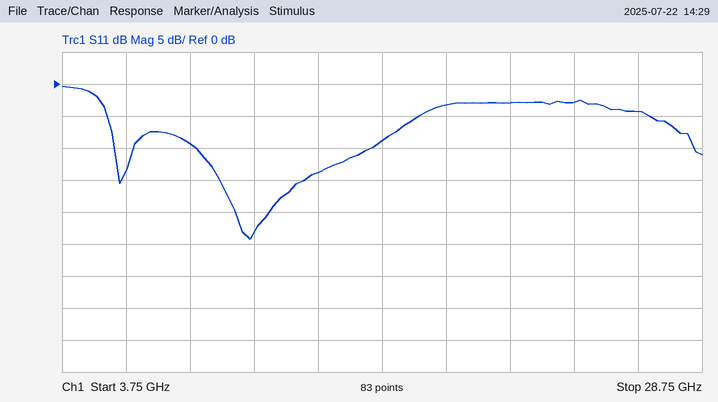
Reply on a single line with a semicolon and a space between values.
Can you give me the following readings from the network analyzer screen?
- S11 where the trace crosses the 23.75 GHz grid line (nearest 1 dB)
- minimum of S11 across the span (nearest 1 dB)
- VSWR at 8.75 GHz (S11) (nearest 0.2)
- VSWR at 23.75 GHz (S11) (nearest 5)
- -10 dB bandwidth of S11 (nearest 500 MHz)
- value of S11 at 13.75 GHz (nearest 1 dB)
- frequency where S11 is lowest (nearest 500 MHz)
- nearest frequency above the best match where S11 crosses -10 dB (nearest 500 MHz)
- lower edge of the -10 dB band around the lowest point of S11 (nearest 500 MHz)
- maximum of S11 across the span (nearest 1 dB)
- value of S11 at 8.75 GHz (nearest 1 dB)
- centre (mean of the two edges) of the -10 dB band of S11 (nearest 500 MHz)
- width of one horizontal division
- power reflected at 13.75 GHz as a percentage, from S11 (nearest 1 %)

-3 dB; -24 dB; 2.0; 5; 7.0 GHz; -14 dB; 11.0 GHz; 16.0 GHz; 9.0 GHz; 0 dB; -9 dB; 12.5 GHz; 2.5 GHz; 4 %
